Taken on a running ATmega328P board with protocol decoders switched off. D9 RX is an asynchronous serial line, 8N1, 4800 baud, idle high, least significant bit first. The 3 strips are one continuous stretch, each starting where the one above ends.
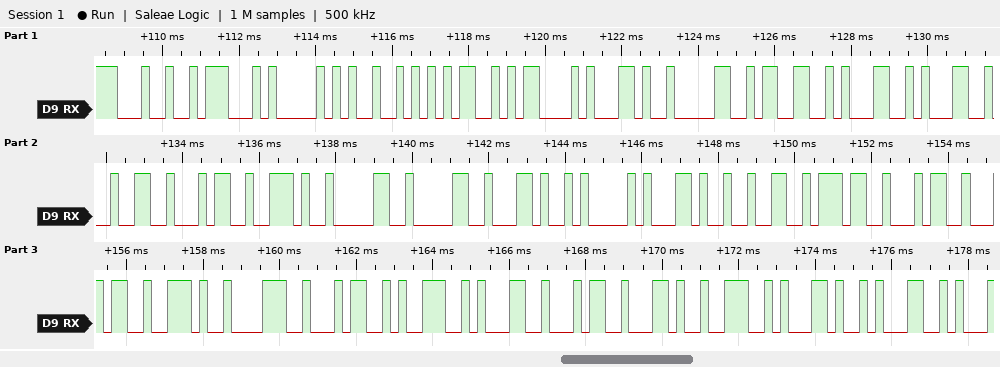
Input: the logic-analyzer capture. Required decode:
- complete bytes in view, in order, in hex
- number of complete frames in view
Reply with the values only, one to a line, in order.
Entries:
24 47 50 52 4D 43 2C 30 33 31 31 32 34 2E 30 30 2C 41 2C 32 37 34 34 2E 38 34 39 31 34 2C 4E 2C 31
33
